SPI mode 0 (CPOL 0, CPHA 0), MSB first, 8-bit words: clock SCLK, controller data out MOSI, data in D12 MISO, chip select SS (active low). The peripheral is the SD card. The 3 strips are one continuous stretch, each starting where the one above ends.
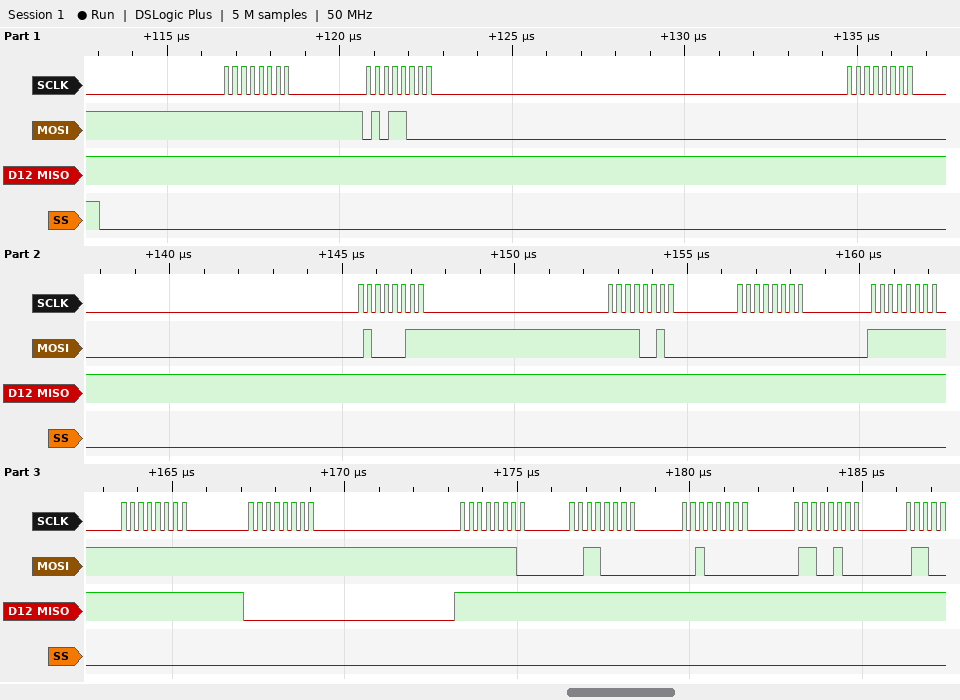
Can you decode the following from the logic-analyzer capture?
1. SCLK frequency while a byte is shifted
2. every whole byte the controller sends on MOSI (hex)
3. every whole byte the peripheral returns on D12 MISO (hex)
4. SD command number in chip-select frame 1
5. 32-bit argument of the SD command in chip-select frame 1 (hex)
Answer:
4 MHz
0xFF 0x58 0x00 0x43 0xF2 0x00 0xFF 0xFF 0xFF 0xFE 0x30 0x20 0x64
0xFF 0xFF 0xFF 0xFF 0xFF 0xFF 0xFF 0xFF 0x00 0xFF 0xFF 0xFF 0xFF
CMD24
0x0043F200
